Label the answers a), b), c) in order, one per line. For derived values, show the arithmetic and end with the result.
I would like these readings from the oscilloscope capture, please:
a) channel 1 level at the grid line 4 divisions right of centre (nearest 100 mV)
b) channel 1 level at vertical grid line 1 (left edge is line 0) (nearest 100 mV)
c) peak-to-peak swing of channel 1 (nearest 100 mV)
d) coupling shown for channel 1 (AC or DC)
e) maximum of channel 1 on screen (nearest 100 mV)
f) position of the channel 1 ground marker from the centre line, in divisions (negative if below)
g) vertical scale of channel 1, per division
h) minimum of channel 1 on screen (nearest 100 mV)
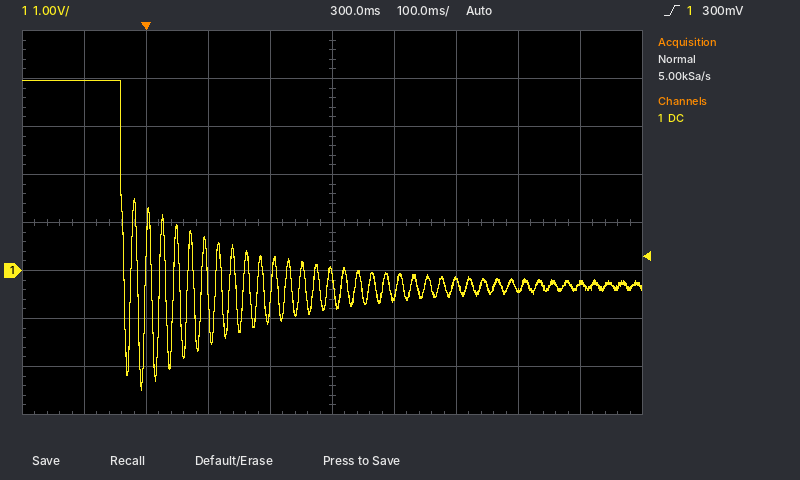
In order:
a) -300 mV
b) 4.0 V
c) 4.0 V − (-2.5 V) = 6.5 V
d) DC
e) 4.0 V
f) -1.0 div
g) 1 V
h) -2.5 V
